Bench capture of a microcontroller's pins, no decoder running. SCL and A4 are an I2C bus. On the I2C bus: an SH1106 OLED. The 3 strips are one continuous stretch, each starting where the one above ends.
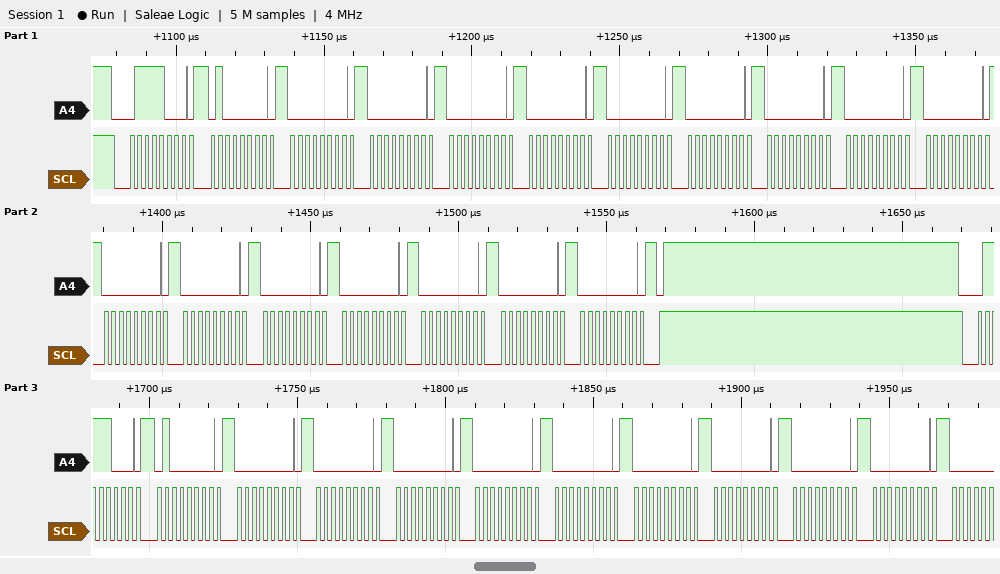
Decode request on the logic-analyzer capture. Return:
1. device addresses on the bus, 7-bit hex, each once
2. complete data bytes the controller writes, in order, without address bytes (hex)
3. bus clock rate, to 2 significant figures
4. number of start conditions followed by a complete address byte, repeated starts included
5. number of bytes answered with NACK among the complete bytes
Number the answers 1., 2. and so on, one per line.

1. 0x3C
2. 40 00 00 00 00 00 00 00 00 00 00 00 00 00 00 00 00 40 00 00 00 00 00 00 00 00 00
3. 400 kHz
4. 2
5. 0
